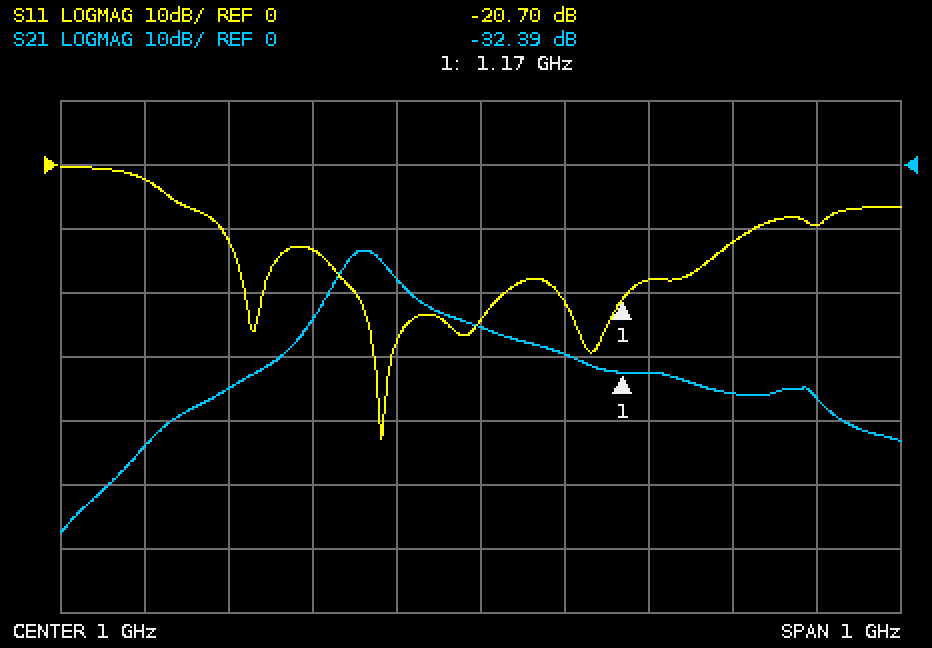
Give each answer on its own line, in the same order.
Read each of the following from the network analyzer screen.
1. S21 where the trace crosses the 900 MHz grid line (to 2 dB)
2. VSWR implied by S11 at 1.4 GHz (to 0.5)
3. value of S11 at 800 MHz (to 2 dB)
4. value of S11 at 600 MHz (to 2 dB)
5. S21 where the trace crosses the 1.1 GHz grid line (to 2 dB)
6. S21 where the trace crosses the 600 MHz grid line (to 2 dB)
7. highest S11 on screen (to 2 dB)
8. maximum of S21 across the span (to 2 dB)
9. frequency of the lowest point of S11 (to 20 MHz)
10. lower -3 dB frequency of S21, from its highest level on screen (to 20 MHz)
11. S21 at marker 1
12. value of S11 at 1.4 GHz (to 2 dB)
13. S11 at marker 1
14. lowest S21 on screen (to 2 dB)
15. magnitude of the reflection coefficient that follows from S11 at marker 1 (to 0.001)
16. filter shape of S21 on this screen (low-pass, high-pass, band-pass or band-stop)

-18 dB
2.0
-14 dB
-2 dB
-30 dB
-44 dB
0 dB
-14 dB
880 MHz
840 MHz
-32.39 dB
-10 dB
-20.70 dB
-58 dB
0.092
band-pass
